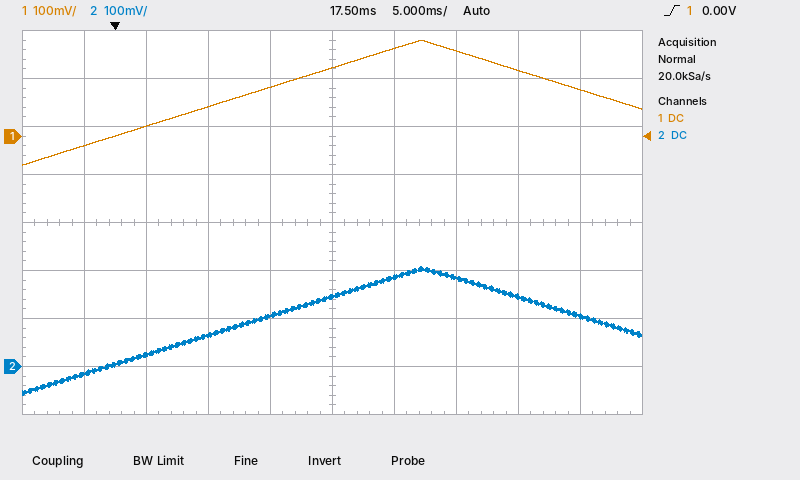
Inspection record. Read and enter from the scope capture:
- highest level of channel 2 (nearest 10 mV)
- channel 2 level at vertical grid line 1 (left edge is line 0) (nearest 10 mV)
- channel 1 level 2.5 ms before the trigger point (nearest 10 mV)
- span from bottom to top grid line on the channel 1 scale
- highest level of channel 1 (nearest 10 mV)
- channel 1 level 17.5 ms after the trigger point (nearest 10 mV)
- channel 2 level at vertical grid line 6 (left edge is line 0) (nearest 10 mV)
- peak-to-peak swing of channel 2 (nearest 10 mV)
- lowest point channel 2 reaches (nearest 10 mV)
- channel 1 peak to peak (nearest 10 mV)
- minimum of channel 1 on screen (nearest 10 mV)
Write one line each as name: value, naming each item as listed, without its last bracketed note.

highest level of channel 2: 210 mV
channel 2 level at vertical grid line 1 (left edge is line 0): -20 mV
channel 1 level 2.5 ms before the trigger point: -20 mV
span from bottom to top grid line on the channel 1 scale: 800 mV
highest level of channel 1: 200 mV
channel 1 level 17.5 ms after the trigger point: 140 mV
channel 2 level at vertical grid line 6 (left edge is line 0): 190 mV
peak-to-peak swing of channel 2: 270 mV
lowest point channel 2 reaches: -60 mV
channel 1 peak to peak: 260 mV
minimum of channel 1 on screen: -60 mV
